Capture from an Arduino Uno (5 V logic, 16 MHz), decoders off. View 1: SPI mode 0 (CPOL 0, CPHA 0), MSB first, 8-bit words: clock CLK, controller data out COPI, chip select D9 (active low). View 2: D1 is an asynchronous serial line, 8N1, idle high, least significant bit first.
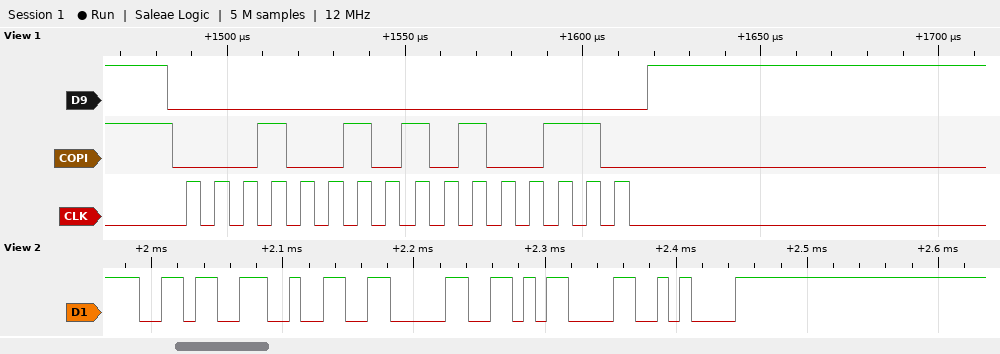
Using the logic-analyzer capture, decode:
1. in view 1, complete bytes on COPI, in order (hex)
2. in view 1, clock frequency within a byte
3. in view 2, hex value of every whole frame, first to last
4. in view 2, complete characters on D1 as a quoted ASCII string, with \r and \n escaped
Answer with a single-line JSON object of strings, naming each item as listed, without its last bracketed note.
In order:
{"in view 1, complete bytes on COPI, in order": "12 A6", "in view 1, clock frequency within a byte": "125 kHz", "in view 2, hex value of every whole frame, first to last": "0x36 0x32 0x30 0x0D 0x0A", "in view 2, complete characters on D1 as a quoted ASCII string, with \\r and \\n escaped": "\"620\\r\\n\""}
